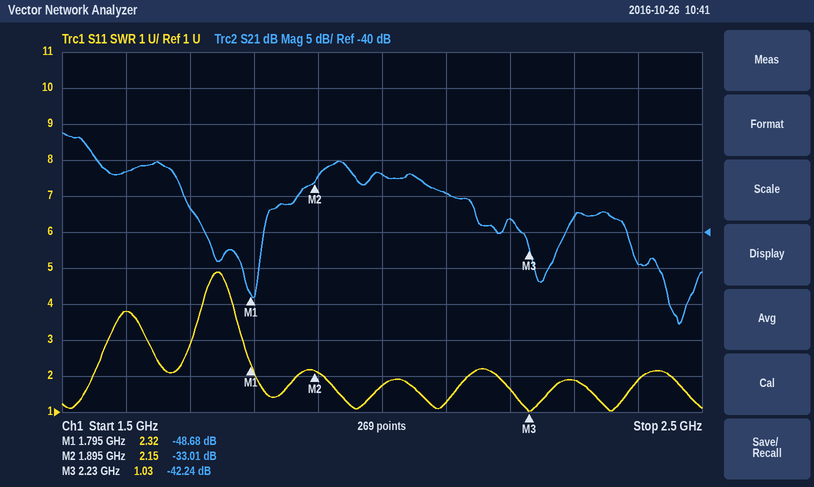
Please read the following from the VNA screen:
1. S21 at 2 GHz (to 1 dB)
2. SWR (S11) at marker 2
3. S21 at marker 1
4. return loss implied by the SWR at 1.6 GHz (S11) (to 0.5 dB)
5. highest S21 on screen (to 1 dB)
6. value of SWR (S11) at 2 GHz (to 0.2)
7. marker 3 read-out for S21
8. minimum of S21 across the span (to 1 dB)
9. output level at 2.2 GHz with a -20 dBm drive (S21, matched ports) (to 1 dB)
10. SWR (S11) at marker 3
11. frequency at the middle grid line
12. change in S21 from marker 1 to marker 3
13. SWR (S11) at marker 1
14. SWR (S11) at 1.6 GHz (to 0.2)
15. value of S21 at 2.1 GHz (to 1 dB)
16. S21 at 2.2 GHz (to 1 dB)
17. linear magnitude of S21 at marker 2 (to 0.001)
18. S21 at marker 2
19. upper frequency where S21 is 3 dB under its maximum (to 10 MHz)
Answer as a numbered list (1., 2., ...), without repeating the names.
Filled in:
1. -32 dB
2. 2.15
3. -48.68 dB
4. 4.5 dB
5. -26 dB
6. 1.8
7. -42.24 dB
8. -53 dB
9. -58 dBm
10. 1.03
11. 2 GHz
12. 6.44 dB
13. 2.32
14. 3.8
15. -35 dB
16. -38 dB
17. 0.022
18. -33.01 dB
19. 1.55 GHz
